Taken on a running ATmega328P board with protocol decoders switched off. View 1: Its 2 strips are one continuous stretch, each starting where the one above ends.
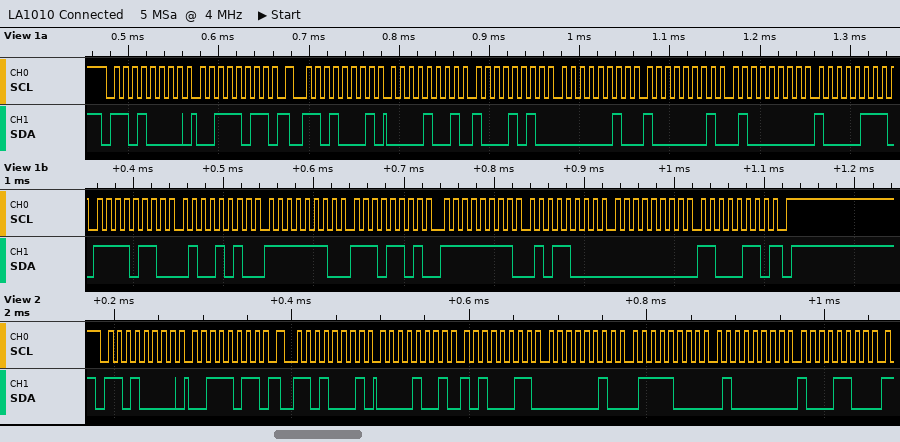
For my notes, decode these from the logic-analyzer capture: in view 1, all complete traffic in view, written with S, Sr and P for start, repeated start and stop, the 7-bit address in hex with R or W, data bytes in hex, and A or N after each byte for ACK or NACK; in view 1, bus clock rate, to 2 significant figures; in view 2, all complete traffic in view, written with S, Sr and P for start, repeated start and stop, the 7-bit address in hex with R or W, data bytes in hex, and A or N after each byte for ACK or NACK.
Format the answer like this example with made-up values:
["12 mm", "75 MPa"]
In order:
["S 68W A 3B A Sr 68R A 09 A 8A A 02 A 81 A 40 A 87 A F6 A 4A A FE A ED A FF A 58 A 00 A C6 N P", "100 kHz", "S 68W A 3B A Sr 68R A 09 A A3 A 02 A 78 A 40 A 8C A"]
